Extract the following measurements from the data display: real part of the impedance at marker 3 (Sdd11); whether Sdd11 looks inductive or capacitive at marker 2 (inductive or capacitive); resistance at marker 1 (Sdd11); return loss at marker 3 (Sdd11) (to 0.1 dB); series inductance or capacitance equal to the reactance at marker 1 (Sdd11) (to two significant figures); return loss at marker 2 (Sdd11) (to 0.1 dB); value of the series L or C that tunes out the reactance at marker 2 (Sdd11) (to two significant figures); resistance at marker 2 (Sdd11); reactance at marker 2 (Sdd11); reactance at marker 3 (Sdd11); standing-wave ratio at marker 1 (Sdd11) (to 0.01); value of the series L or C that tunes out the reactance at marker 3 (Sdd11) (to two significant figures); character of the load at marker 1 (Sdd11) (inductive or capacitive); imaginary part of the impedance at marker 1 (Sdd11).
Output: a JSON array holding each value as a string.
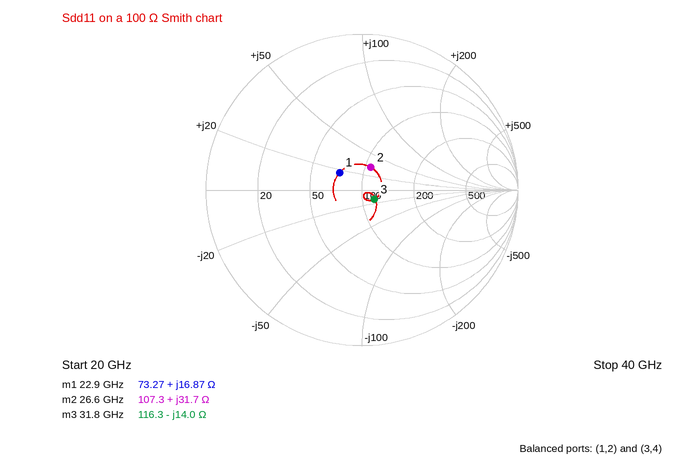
["116.3 Ω", "inductive", "73.27 Ω", "20.1 dB", "120 pH", "16.2 dB", "190 fF", "107.3 Ω", "+31.7 Ω", "-14.0 Ω", "1.44", "70 pH", "inductive", "+16.87 Ω"]
